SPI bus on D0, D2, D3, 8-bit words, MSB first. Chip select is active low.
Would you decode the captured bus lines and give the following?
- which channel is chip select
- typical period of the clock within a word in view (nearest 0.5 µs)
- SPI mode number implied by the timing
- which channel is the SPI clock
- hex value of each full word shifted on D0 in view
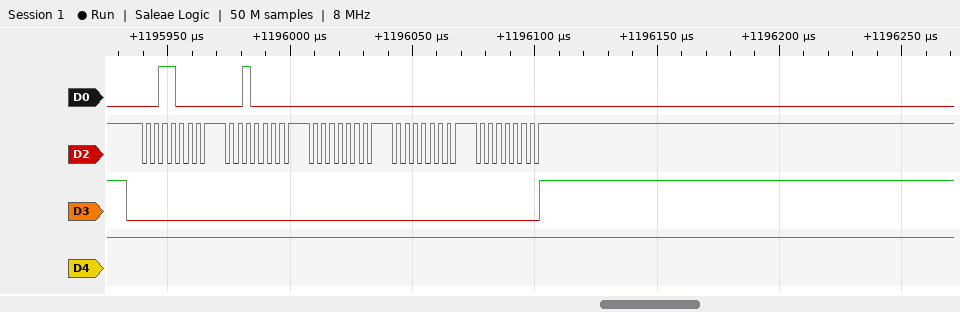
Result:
D3
3.5 µs
3
D2
30, 20, 00, 00, 00
